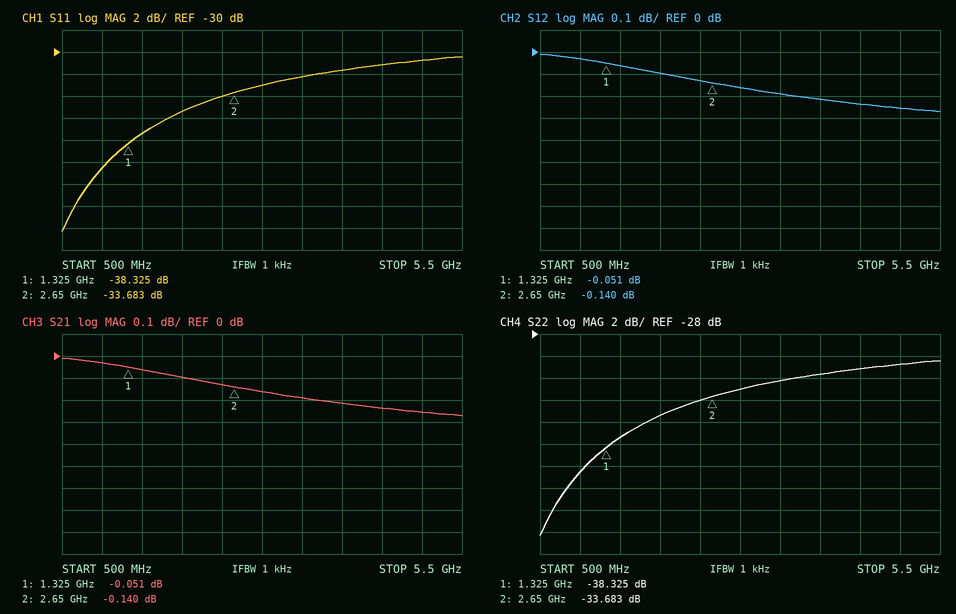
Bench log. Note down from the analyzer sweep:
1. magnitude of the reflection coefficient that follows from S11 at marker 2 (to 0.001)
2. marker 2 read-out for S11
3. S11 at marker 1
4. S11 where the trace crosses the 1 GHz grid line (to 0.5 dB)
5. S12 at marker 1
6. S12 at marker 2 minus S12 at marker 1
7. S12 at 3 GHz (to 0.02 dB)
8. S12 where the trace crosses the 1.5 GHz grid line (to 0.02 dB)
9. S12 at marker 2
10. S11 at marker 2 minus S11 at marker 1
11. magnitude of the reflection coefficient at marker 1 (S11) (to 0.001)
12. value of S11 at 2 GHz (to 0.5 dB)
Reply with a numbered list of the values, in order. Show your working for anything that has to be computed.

1. 10^(-33.683/20) ≈ 0.021
2. -33.683 dB
3. -38.325 dB
4. -40.5 dB
5. -0.051 dB
6. -0.14 − (-0.051) = -0.089 dB
7. -0.16 dB
8. -0.06 dB
9. -0.140 dB
10. -33.683 − (-38.325) = 4.642 dB
11. 10^(-38.325/20) ≈ 0.012
12. -35.5 dB
